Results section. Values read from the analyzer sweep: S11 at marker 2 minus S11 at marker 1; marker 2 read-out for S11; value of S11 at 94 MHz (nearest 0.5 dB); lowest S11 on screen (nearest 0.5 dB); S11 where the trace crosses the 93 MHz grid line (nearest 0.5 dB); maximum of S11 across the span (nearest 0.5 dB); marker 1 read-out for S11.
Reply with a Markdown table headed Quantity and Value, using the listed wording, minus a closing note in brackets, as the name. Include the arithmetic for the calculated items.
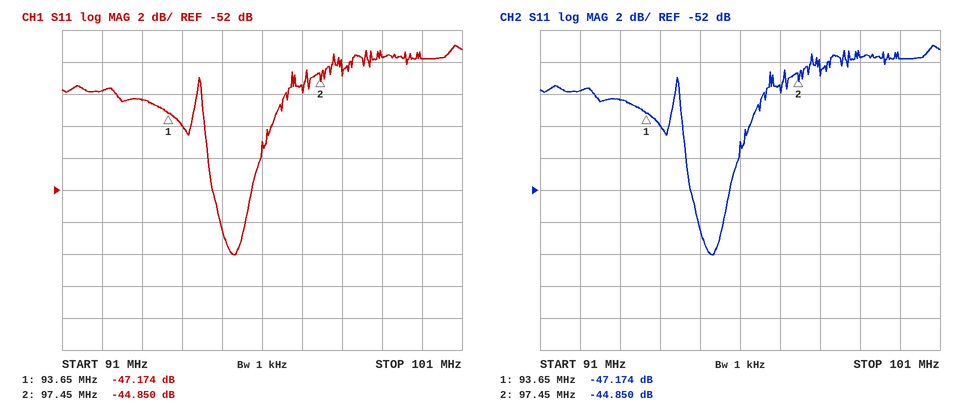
| Quantity | Value |
|---|---|
| S11 at marker 2 minus S11 at marker 1 | -44.85 − (-47.174) = 2.324 dB |
| marker 2 read-out for S11 | -44.850 dB |
| value of S11 at 94 MHz | -48.0 dB |
| lowest S11 on screen | -56.0 dB |
| S11 where the trace crosses the 93 MHz grid line | -46.5 dB |
| maximum of S11 across the span | -43.0 dB |
| marker 1 read-out for S11 | -47.174 dB |
